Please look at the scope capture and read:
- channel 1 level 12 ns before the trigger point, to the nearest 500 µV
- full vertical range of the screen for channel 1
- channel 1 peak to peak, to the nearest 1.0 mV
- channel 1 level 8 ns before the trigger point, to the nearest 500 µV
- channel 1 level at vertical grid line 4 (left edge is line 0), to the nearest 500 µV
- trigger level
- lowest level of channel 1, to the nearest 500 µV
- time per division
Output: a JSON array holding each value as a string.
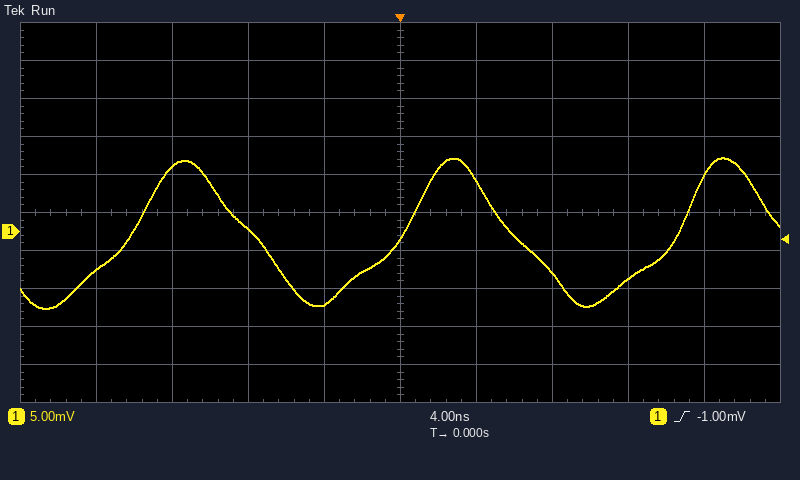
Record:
["8.5 mV", "50 mV", "20.0 mV", "500 µV", "-9.5 mV", "-1.00 mV", "-10.0 mV", "4 ns"]
